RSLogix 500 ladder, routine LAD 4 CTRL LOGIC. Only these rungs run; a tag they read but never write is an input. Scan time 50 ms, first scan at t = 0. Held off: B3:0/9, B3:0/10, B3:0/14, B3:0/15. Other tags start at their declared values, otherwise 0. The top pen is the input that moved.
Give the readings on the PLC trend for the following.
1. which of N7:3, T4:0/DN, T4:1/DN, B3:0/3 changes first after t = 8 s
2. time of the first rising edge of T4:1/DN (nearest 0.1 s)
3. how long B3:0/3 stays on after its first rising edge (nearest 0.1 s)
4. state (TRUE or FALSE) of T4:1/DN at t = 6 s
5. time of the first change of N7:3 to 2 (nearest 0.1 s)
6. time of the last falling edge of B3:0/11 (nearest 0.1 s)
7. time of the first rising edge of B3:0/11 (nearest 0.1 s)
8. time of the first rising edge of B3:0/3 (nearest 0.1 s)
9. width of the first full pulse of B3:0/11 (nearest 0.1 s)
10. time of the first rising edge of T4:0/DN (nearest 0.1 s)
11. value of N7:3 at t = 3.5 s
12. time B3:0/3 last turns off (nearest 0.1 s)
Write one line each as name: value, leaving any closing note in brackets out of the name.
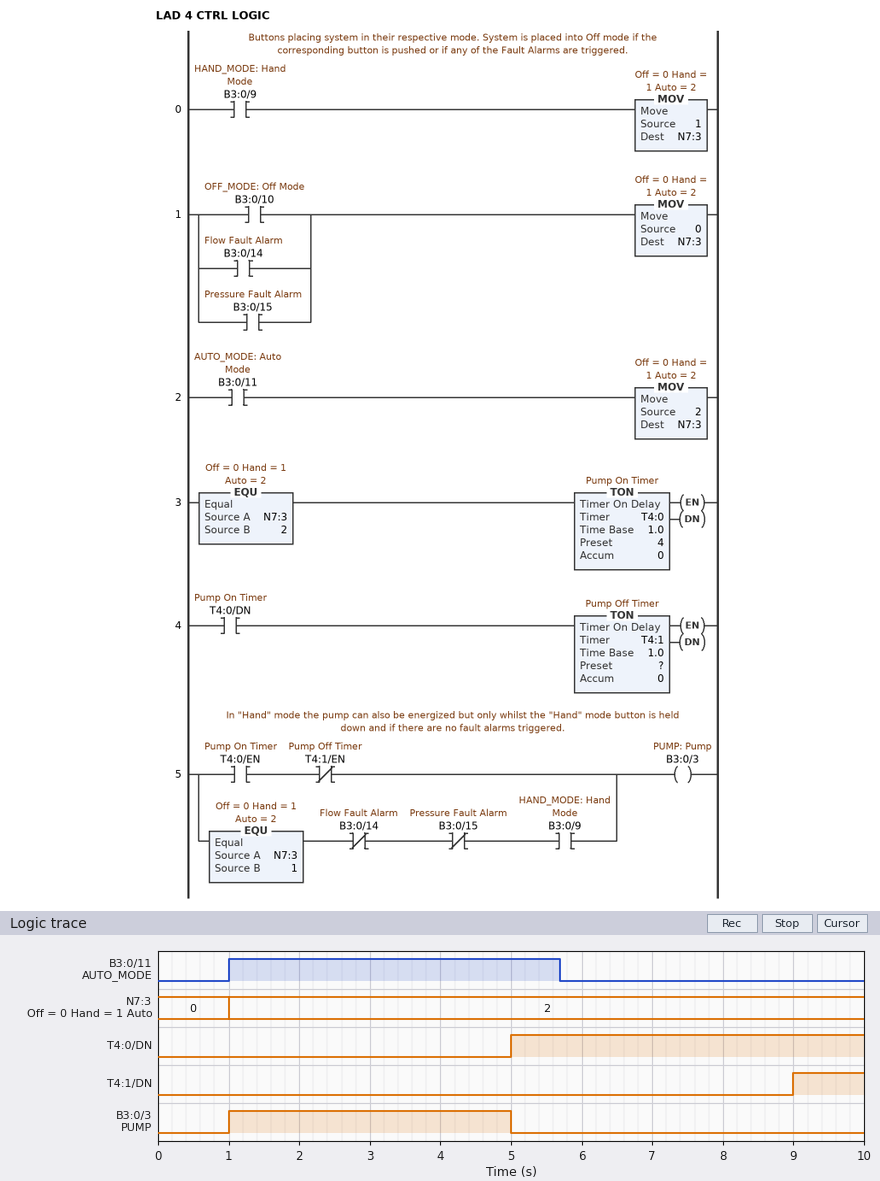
which of N7:3, T4:0/DN, T4:1/DN, B3:0/3 changes first after t = 8 s: T4:1/DN
time of the first rising edge of T4:1/DN: 9.0 s
how long B3:0/3 stays on after its first rising edge: 4.0 s
state (TRUE or FALSE) of T4:1/DN at t = 6 s: FALSE
time of the first change of N7:3 to 2: 1.0 s
time of the last falling edge of B3:0/11: 5.7 s
time of the first rising edge of B3:0/11: 1.0 s
time of the first rising edge of B3:0/3: 1.0 s
width of the first full pulse of B3:0/11: 4.7 s
time of the first rising edge of T4:0/DN: 5.0 s
value of N7:3 at t = 3.5 s: 2
time B3:0/3 last turns off: 5.0 s
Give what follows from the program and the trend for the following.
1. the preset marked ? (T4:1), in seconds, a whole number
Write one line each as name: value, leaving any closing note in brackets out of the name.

the preset marked ? (T4:1), in seconds, a whole number: 4 s
